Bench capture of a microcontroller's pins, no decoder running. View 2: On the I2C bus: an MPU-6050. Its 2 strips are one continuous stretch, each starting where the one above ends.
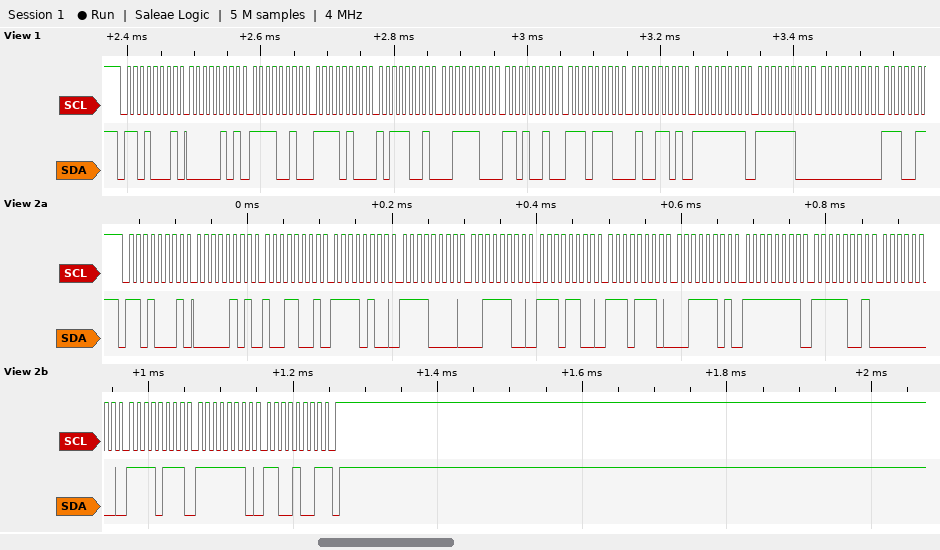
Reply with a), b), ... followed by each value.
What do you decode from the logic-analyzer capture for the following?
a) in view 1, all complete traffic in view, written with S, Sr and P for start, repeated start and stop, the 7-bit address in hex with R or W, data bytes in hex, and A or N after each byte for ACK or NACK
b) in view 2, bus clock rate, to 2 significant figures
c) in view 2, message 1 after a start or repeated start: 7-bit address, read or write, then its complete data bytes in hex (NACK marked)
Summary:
a) S 68R A 05 A F2 A F4 A B9 A 3C A D2 A EE A 4D A FF A FC A 00 A
b) 100 kHz
c) 0x68 read: 05 99 F4 F0 3C EC EE 3D FF F9 00 F7 FE C9 NACK
